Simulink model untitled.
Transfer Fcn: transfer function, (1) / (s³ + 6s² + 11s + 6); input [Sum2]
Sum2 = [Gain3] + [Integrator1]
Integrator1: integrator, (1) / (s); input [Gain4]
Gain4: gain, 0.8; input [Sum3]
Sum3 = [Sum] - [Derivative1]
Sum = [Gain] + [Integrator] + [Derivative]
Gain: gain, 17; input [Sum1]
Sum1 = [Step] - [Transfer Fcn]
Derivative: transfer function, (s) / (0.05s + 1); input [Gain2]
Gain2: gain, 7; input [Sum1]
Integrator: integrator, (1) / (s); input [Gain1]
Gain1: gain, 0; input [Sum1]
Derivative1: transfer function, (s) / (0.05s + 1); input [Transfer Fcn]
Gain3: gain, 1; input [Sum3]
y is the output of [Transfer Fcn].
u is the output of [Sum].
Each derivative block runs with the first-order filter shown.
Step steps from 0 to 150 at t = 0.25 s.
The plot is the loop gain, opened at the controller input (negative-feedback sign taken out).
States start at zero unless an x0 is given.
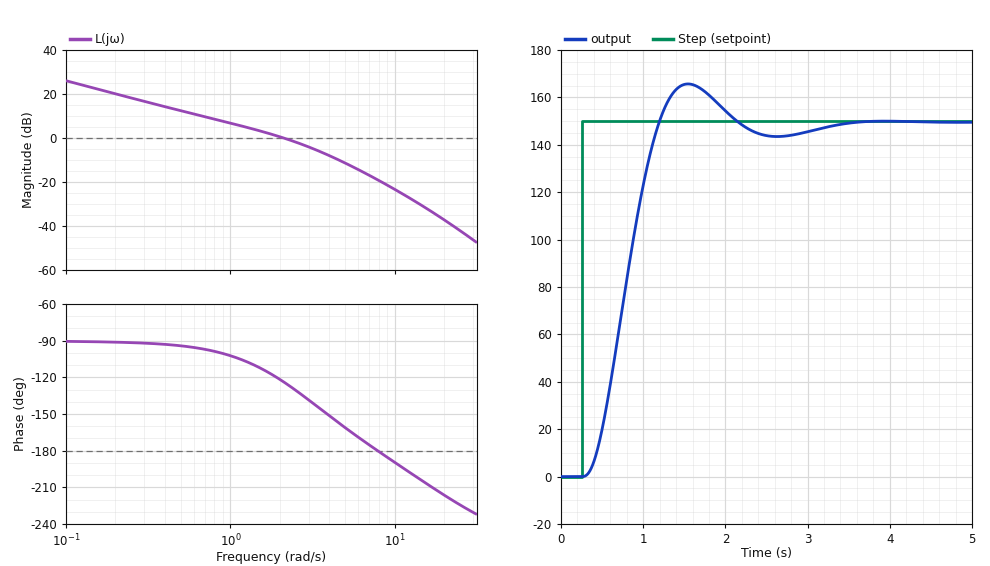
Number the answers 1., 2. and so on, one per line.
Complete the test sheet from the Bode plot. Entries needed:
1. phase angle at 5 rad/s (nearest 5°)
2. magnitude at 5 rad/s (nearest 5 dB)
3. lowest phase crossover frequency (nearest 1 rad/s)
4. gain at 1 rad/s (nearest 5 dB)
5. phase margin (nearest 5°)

1. -160°
2. -10 dB
3. 8 rad/s
4. 5 dB
5. 55°
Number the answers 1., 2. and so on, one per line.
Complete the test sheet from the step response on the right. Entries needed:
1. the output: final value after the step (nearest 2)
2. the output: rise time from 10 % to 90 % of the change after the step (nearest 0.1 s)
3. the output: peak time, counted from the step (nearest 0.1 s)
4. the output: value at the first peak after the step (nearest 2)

1. 150
2. 0.6 s
3. 1.3 s
4. 166
